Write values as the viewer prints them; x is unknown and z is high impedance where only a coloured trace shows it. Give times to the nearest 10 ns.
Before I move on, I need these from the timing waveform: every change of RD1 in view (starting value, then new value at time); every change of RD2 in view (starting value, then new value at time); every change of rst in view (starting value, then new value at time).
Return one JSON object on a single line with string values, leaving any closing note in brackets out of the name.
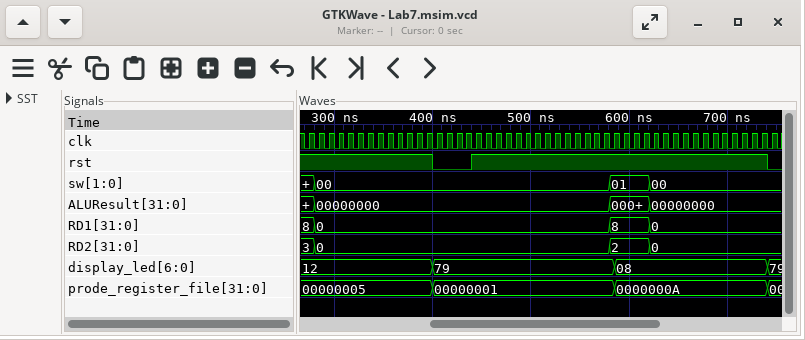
{"every change of RD1 in view": "8, 0 at 280 ns, 8 at 580 ns, 0 at 620 ns", "every change of RD2 in view": "3, 0 at 280 ns, 2 at 580 ns, 0 at 620 ns", "every change of rst in view": "1, 0 at 400 ns, 1 at 440 ns, 0 at 740 ns"}
